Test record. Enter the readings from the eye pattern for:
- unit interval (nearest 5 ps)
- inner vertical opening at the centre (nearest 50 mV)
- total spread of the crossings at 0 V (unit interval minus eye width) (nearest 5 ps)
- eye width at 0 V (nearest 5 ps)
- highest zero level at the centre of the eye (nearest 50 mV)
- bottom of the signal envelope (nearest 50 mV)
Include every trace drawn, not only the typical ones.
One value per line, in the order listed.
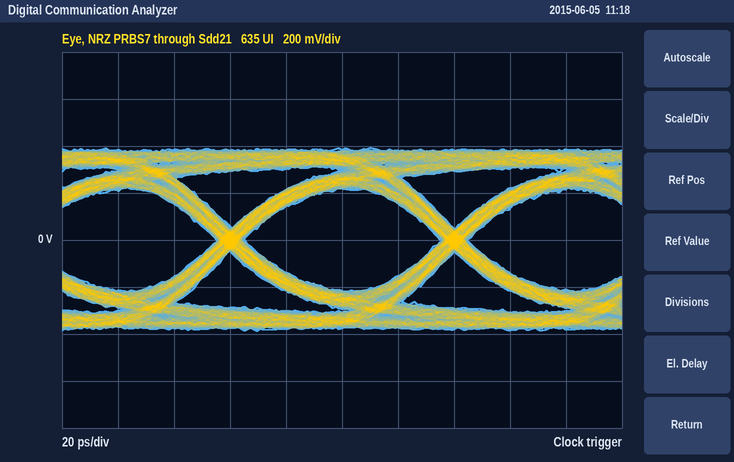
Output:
80 ps
450 mV
10 ps
70 ps
-200 mV
-400 mV
